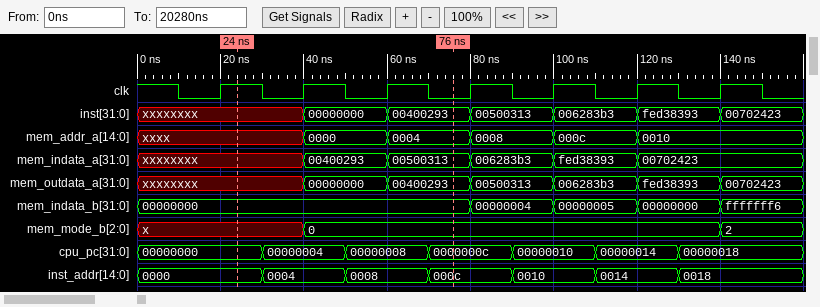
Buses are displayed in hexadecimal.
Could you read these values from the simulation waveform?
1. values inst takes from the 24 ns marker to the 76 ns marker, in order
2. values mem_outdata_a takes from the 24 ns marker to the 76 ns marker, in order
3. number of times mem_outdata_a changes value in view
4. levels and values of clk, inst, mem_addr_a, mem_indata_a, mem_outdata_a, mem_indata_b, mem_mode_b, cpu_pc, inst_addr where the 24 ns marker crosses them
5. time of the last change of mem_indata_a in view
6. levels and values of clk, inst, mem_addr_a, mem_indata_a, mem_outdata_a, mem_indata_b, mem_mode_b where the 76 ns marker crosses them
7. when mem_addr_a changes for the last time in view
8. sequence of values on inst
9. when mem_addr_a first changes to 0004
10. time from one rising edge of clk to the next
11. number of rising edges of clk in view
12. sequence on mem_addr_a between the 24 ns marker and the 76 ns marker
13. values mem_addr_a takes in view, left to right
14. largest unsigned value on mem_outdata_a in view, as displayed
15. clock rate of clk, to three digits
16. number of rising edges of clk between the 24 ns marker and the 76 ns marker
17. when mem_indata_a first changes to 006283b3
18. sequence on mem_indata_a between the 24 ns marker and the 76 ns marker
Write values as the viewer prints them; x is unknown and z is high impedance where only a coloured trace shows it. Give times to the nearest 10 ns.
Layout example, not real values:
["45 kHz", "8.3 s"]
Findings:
["xxxxxxxx, 00000000, 00400293", "xxxxxxxx, 00000000, 00400293", "6", "clk=1, inst=xxxxxxxx, mem_addr_a=xxxx, mem_indata_a=xxxxxxxx, mem_outdata_a=xxxxxxxx, mem_indata_b=00000000, mem_mode_b=x, cpu_pc=00000000, inst_addr=0000", "120 ns", "clk=0, inst=00400293, mem_addr_a=0004, mem_indata_a=00500313, mem_outdata_a=00400293, mem_indata_b=00000000, mem_mode_b=0", "120 ns", "xxxxxxxx, 00000000, 00400293, 00500313, 006283b3, fed38393, 00702423", "60 ns", "20 ns", "7", "xxxx, 0000, 0004", "xxxx, 0000, 0004, 0008, 000c, 0010", "fed38393", "50.0 MHz", "2", "80 ns", "xxxxxxxx, 00400293, 00500313"]
